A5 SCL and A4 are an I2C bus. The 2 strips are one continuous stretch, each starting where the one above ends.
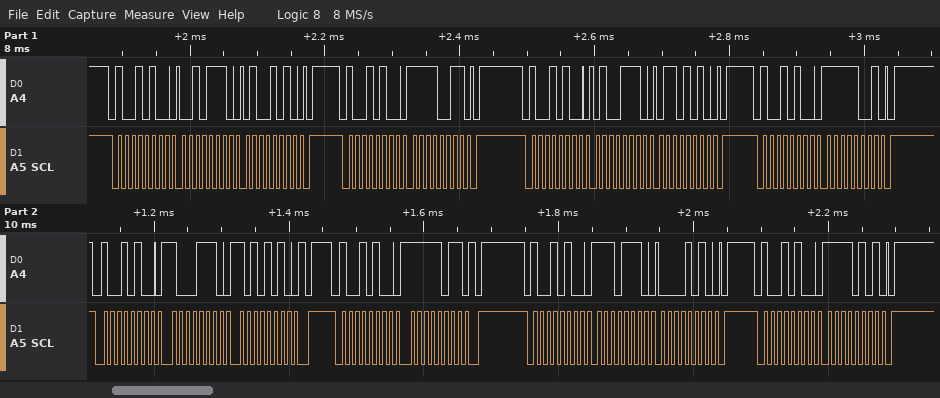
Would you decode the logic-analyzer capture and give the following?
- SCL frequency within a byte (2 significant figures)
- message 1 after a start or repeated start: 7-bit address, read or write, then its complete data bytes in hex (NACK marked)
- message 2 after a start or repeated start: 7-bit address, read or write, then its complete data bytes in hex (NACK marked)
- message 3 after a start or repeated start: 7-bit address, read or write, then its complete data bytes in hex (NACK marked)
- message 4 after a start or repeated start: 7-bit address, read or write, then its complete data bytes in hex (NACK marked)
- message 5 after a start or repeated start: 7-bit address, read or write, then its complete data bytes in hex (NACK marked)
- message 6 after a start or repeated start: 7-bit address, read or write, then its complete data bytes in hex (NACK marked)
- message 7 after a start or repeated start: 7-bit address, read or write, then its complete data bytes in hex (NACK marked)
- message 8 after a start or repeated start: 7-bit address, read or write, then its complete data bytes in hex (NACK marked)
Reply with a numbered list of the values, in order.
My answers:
1. 100 kHz
2. 0x4A write: 2E 4A
3. 0x4A write: F3
4. 0x4A write: 4E 6A
5. 0x4A write: F9
6. 0x4A write: 8E AA
7. 0x4A write: FB
8. 0x4A write: EE 0A
9. 0x4A write: F5
